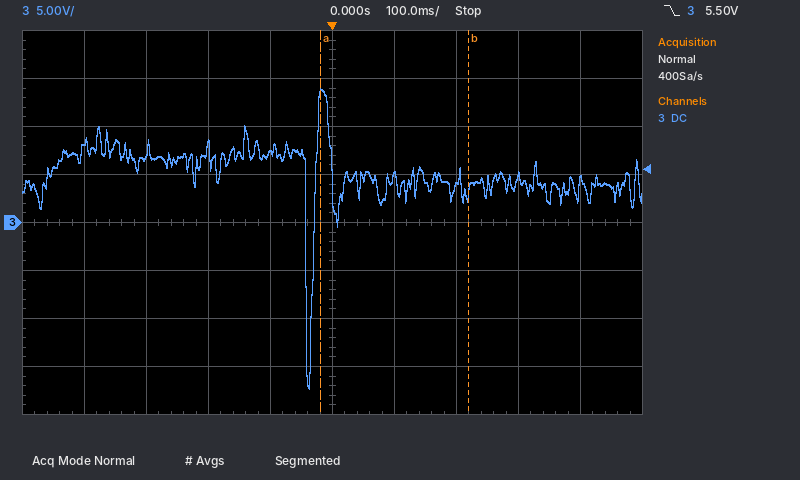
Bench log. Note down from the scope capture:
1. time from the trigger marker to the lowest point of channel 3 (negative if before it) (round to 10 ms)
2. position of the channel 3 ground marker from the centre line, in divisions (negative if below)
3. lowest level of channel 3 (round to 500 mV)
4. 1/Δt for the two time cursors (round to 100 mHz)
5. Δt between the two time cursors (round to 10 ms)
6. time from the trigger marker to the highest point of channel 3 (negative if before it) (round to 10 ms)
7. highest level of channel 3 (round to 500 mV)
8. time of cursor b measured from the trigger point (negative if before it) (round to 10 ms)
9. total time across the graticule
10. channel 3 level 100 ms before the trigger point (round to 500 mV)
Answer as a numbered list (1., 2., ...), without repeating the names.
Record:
1. -40 ms
2. 0.0 div
3. -17.5 V
4. 4.2 Hz
5. 240 ms
6. -20 ms
7. 14.0 V
8. +220 ms
9. 1 s
10. 7.0 V
